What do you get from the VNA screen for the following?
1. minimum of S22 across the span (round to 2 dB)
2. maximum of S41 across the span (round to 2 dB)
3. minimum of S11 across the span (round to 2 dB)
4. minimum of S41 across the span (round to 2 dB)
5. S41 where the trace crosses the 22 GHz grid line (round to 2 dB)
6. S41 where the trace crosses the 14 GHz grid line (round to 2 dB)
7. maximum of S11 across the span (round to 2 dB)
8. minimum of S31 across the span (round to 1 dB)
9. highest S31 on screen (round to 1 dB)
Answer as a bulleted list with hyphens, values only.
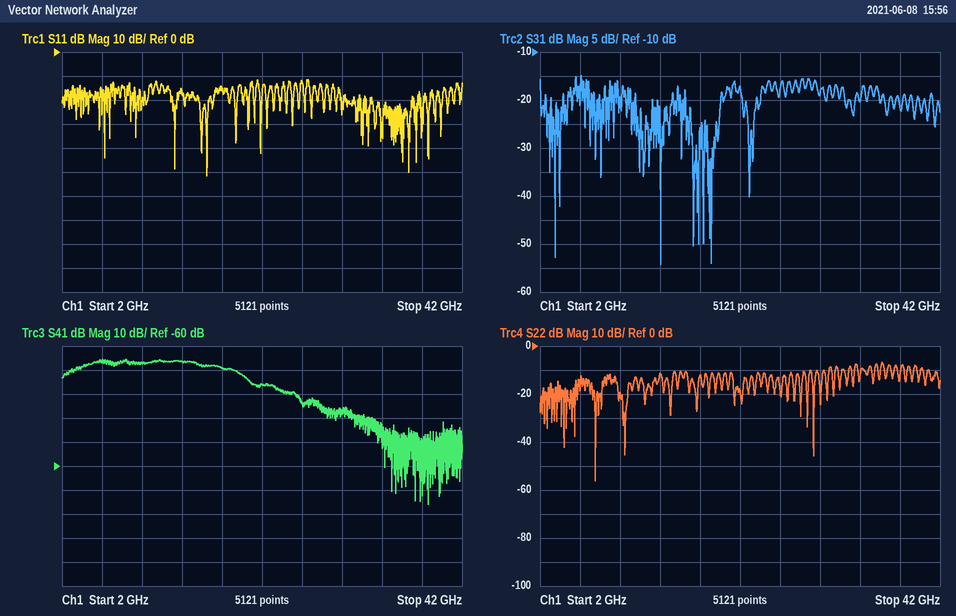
- -56 dB
- -16 dB
- -52 dB
- -76 dB
- -26 dB
- -16 dB
- -12 dB
- -54 dB
- -15 dB
